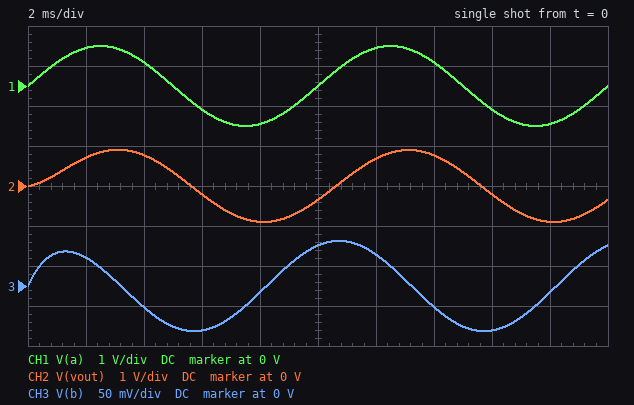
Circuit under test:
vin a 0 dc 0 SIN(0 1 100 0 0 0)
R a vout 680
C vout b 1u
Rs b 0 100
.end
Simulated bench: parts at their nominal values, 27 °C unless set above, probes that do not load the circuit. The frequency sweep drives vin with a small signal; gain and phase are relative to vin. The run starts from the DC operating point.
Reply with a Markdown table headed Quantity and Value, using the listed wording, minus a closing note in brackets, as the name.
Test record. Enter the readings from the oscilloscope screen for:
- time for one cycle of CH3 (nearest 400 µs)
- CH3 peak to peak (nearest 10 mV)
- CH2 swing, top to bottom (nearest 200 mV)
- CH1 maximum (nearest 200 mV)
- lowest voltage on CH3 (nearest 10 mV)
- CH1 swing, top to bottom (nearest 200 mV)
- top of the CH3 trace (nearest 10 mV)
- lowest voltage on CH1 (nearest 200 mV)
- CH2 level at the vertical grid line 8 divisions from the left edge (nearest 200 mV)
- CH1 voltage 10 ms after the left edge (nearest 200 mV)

| Quantity | Value |
|---|---|
| time for one cycle of CH3 | 10.0 ms |
| CH3 peak to peak | 110 mV |
| CH2 swing, top to bottom | 1.8 V |
| CH1 maximum | 1.0 V |
| lowest voltage on CH3 | -60 mV |
| CH1 swing, top to bottom | 2.0 V |
| top of the CH3 trace | 60 mV |
| lowest voltage on CH1 | -1.0 V |
| CH2 level at the vertical grid line 8 divisions from the left edge | -200 mV |
| CH1 voltage 10 ms after the left edge | 0 V |
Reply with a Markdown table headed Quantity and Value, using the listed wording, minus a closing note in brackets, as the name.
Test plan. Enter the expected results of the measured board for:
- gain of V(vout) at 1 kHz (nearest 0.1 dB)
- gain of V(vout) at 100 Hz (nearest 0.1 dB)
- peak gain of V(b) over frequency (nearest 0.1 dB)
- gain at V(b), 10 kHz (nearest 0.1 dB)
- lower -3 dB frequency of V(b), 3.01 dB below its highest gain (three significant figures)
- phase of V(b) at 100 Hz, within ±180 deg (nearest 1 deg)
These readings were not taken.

| Quantity | Value |
|---|---|
| gain of V(vout) at 1 kHz | -12.5 dB |
| gain of V(vout) at 100 Hz | -0.9 dB |
| peak gain of V(b) over frequency | -17.8 dB |
| gain at V(b), 10 kHz | -17.8 dB |
| lower -3 dB frequency of V(b), 3.01 dB below its highest gain | 204 Hz |
| phase of V(b) at 100 Hz, within ±180 deg | 64 deg |
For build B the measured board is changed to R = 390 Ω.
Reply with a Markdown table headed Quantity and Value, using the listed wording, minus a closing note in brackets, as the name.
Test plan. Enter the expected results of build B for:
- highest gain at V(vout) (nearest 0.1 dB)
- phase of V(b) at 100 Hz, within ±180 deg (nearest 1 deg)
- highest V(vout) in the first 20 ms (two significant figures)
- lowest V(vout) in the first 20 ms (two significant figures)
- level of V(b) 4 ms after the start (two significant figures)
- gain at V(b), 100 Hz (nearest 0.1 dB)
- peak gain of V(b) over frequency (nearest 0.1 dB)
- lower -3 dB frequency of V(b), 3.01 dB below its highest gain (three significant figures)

| Quantity | Value |
|---|---|
| highest gain at V(vout) | 0 dB |
| phase of V(b) at 100 Hz, within ±180 deg | 73 deg |
| highest V(vout) in the first 20 ms | 960 mV |
| lowest V(vout) in the first 20 ms | -960 mV |
| level of V(b) 4 ms after the start | -36 mV |
| gain at V(b), 100 Hz | -24.4 dB |
| peak gain of V(b) over frequency | -13.8 dB |
| lower -3 dB frequency of V(b), 3.01 dB below its highest gain | 325 Hz |
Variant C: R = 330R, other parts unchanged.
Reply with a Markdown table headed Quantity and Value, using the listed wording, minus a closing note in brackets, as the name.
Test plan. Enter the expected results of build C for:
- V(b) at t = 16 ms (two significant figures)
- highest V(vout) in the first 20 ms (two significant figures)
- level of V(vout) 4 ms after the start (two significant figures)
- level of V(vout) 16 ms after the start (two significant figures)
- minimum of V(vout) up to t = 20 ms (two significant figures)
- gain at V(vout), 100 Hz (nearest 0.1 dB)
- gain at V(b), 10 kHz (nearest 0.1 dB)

| Quantity | Value |
|---|---|
| V(b) at t = 16 ms | -57 mV |
| highest V(vout) in the first 20 ms | 970 mV |
| level of V(vout) 4 ms after the start | 710 mV |
| level of V(vout) 16 ms after the start | -400 mV |
| minimum of V(vout) up to t = 20 ms | -970 mV |
| gain at V(vout), 100 Hz | -0.3 dB |
| gain at V(b), 10 kHz | -12.7 dB |
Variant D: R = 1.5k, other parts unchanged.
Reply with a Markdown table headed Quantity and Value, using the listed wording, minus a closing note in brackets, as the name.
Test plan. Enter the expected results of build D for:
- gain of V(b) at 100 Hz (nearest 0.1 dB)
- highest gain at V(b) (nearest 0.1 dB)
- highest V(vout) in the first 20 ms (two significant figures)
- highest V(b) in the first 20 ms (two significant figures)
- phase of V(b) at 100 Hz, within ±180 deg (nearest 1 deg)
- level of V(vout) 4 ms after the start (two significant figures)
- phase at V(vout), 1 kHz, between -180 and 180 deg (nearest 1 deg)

| Quantity | Value |
|---|---|
| gain of V(b) at 100 Hz | -27.1 dB |
| highest gain at V(b) | -24.1 dB |
| highest V(vout) in the first 20 ms | 760 mV |
| highest V(b) in the first 20 ms | 44 mV |
| phase of V(b) at 100 Hz, within ±180 deg | 45 deg |
| level of V(vout) 4 ms after the start | 730 mV |
| phase at V(vout), 1 kHz, between -180 and 180 deg | -52 deg |
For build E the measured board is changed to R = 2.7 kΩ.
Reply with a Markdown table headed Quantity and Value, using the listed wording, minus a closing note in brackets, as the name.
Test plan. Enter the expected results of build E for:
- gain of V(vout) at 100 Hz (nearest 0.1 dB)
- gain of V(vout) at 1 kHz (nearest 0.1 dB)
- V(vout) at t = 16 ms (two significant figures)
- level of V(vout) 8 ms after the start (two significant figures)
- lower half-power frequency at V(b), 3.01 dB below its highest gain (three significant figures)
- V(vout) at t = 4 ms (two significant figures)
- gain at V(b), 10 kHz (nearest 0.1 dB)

| Quantity | Value |
|---|---|
| gain of V(vout) at 100 Hz | -6.1 dB |
| gain of V(vout) at 1 kHz | -23.5 dB |
| V(vout) at t = 16 ms | 180 mV |
| level of V(vout) 8 ms after the start | -360 mV |
| lower half-power frequency at V(b), 3.01 dB below its highest gain | 56.8 Hz |
| V(vout) at t = 4 ms | 590 mV |
| gain at V(b), 10 kHz | -28.9 dB |
